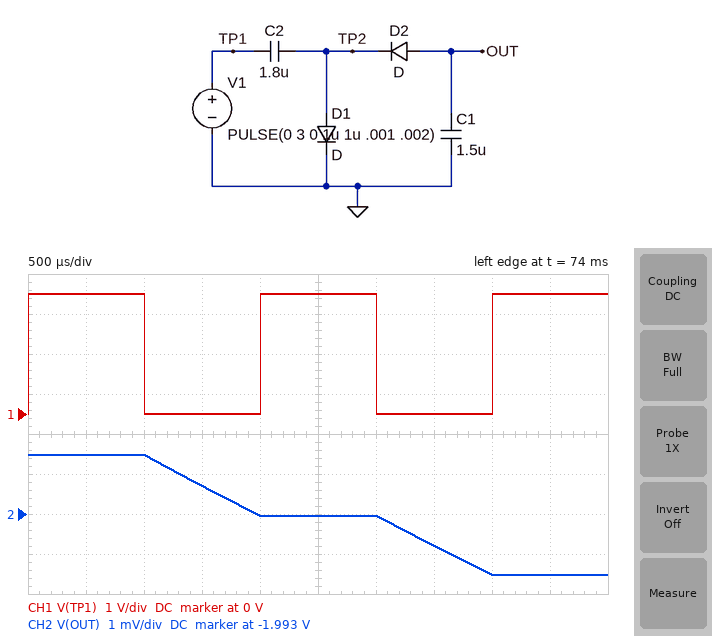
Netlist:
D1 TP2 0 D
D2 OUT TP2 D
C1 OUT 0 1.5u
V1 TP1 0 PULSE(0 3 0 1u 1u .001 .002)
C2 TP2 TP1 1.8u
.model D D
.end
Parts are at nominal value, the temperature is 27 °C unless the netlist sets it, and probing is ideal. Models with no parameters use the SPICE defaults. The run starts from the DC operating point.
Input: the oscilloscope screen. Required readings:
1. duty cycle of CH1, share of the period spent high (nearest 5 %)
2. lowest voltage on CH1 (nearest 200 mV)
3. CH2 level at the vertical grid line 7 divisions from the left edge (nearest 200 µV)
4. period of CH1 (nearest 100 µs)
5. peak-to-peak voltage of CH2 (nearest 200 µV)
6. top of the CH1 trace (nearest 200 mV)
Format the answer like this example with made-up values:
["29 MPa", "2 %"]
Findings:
["50 %", "0 V", "-1.9938 V", "2.0 ms", "3.0 mV", "3.0 V"]
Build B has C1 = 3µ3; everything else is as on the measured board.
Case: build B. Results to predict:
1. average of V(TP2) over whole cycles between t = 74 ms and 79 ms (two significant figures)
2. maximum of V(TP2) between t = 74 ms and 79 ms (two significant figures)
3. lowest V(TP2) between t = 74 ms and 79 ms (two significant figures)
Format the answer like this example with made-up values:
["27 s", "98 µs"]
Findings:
["-970 mV", "530 mV", "-2.5 V"]
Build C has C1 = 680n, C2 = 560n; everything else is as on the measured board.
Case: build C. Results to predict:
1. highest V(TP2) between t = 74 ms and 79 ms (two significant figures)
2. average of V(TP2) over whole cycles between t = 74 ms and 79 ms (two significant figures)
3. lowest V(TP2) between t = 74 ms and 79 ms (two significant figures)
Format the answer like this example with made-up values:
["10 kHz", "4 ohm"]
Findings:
["490 mV", "-1.0 V", "-2.5 V"]
